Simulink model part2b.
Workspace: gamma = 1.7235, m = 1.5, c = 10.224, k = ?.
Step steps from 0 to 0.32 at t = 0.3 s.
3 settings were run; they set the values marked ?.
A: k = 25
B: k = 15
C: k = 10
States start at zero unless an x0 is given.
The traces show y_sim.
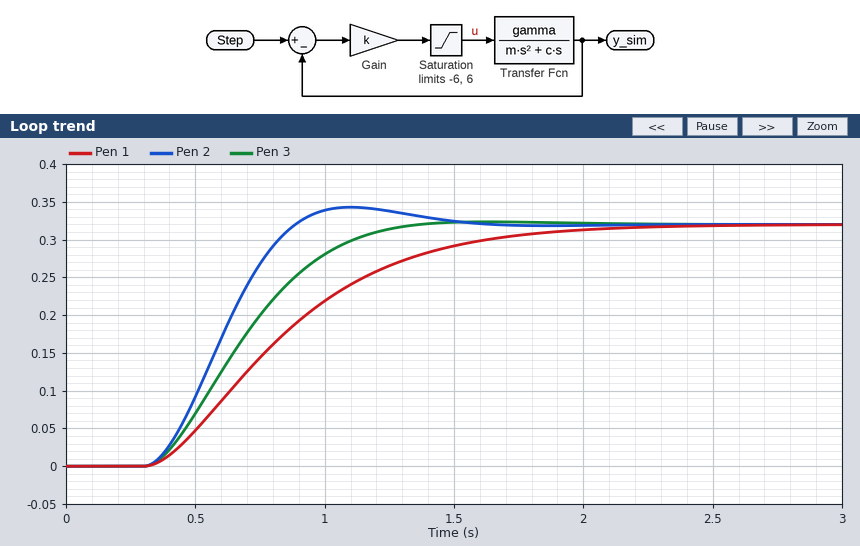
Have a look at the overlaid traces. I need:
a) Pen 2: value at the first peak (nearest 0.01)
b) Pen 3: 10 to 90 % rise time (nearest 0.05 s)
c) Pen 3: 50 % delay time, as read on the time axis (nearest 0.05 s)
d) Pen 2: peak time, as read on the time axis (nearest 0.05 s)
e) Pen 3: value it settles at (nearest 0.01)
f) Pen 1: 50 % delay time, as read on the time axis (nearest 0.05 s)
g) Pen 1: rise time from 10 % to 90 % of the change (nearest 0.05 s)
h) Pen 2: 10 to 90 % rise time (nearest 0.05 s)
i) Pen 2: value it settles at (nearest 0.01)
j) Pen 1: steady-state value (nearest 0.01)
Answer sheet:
0.34
0.60 s
0.65 s
1.10 s
0.32
0.80 s
1.00 s
0.40 s
0.32
0.32
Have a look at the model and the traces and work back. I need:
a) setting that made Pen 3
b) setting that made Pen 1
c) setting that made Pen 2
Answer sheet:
B
C
A
